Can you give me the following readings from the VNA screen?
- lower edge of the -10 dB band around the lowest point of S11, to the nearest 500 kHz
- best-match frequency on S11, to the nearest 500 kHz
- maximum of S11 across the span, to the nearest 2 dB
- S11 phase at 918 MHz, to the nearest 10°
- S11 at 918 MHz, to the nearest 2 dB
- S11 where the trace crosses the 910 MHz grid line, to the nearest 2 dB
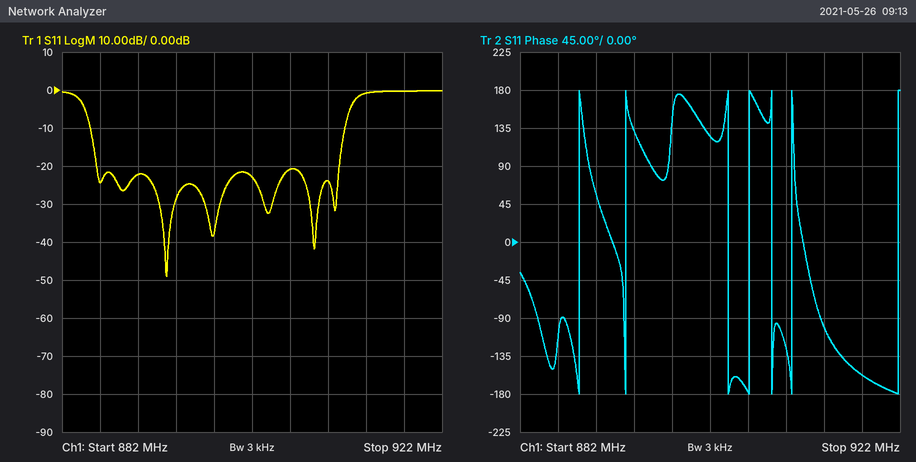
885.0 MHz
893.0 MHz
0 dB
-160°
0 dB
-24 dB
